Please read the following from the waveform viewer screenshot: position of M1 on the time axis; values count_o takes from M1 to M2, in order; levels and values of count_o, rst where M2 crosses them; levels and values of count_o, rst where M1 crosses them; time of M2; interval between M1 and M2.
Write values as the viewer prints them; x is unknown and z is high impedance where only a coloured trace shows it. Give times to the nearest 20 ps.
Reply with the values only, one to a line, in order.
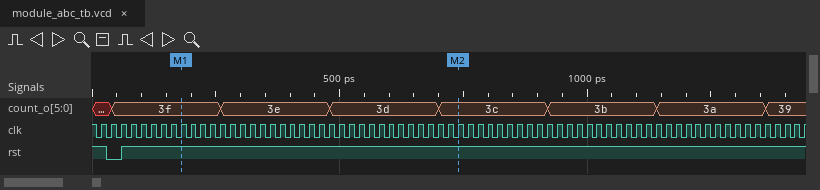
180 ps
3f, 3e, 3d, 3c
count_o=3c, rst=1
count_o=3f, rst=1
740 ps
560 ps
